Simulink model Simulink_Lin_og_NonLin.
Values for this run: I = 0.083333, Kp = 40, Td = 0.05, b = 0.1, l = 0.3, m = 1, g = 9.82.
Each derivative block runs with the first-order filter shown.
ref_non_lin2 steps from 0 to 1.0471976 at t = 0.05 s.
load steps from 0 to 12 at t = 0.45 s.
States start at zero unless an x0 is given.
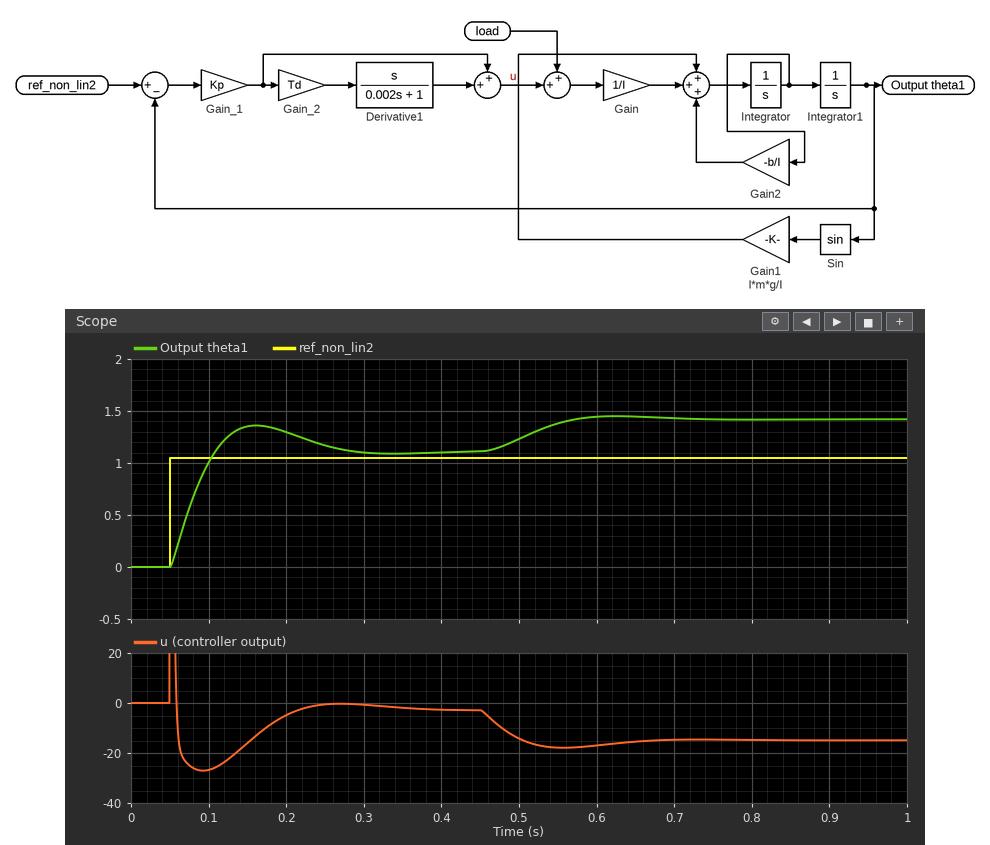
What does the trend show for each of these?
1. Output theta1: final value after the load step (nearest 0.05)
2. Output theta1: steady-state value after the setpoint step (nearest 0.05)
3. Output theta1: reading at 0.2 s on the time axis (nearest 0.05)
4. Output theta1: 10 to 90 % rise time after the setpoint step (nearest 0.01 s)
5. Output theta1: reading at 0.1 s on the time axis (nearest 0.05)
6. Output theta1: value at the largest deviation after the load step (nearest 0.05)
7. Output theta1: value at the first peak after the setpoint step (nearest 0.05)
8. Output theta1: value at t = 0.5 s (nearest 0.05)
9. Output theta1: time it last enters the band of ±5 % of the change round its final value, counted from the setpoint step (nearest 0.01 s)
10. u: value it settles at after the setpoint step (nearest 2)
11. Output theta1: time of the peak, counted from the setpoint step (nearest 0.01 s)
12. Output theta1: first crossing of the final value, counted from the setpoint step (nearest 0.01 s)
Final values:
1.40
1.10
1.30
0.04 s
1.00
1.45
1.35
1.25
0.20 s
-2
0.11 s
0.06 s
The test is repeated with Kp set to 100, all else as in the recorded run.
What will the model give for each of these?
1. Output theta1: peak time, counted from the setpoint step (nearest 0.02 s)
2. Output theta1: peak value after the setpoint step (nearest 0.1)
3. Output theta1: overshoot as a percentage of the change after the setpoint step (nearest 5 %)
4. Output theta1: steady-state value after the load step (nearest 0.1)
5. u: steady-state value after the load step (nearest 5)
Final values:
0.06 s
1.2
15 %
1.2
-15
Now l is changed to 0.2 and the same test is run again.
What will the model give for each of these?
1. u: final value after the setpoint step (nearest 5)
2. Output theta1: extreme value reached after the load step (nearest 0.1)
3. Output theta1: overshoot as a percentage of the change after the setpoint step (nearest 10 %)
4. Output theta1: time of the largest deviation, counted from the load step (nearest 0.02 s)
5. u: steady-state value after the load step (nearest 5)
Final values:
0
1.4
20 %
0.18 s
-15
